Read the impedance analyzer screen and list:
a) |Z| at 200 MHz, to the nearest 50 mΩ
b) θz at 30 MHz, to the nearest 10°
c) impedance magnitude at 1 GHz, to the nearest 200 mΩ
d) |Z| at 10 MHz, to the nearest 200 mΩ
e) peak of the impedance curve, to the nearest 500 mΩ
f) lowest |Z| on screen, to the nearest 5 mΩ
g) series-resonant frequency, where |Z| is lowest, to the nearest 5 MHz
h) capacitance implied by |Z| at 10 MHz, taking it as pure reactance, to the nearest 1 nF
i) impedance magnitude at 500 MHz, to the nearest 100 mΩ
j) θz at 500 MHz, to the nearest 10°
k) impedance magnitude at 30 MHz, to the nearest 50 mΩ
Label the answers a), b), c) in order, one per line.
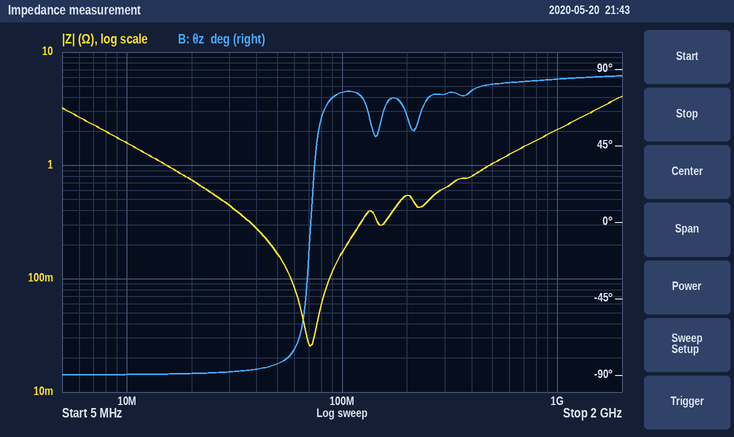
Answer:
a) 550 mΩ
b) -90°
c) 2.0 Ω
d) 1.6 Ω
e) 4.0 Ω
f) 25 mΩ
g) 70 MHz
h) 10 nF
i) 1.0 Ω
j) 80°
k) 450 mΩ
